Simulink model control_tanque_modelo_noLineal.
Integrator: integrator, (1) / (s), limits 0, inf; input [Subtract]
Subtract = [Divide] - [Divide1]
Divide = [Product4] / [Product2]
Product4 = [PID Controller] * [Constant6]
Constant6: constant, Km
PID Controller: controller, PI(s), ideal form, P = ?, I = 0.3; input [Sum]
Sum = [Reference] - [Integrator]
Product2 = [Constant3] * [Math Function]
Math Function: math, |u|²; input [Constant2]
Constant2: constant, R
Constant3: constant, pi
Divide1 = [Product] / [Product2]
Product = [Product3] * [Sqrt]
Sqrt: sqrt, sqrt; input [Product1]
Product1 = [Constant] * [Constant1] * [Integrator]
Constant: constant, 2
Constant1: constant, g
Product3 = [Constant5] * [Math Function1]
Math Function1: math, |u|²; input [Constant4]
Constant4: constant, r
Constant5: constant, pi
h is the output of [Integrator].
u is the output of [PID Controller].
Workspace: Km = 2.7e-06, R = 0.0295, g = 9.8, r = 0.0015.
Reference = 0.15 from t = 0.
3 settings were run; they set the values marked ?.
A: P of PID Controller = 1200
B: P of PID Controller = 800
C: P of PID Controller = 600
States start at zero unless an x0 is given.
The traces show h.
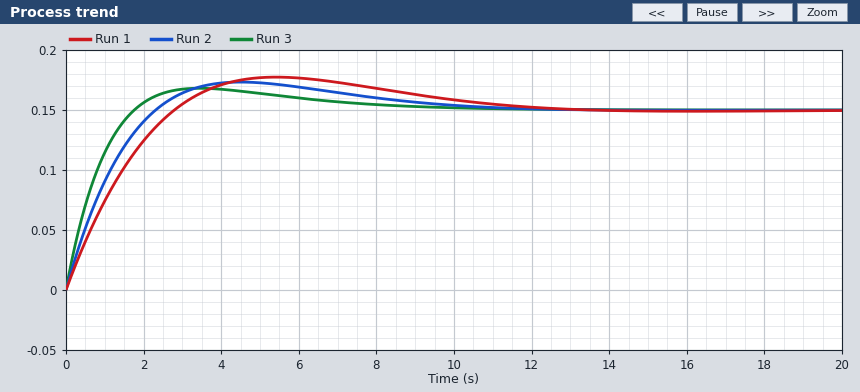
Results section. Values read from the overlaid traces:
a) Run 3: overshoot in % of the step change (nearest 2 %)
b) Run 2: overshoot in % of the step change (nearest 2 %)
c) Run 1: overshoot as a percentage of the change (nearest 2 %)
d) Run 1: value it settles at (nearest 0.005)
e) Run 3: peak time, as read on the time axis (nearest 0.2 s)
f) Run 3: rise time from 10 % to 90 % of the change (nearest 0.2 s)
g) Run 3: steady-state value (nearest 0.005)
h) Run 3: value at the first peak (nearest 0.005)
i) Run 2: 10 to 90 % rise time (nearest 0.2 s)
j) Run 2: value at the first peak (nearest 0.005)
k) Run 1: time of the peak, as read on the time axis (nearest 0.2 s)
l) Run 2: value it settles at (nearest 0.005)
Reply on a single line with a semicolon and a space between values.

12 %; 16 %; 18 %; 0.150; 3.4 s; 1.2 s; 0.150; 0.170; 1.8 s; 0.175; 5.4 s; 0.150
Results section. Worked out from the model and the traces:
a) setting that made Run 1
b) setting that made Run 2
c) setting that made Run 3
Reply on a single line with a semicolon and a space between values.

C; B; A
